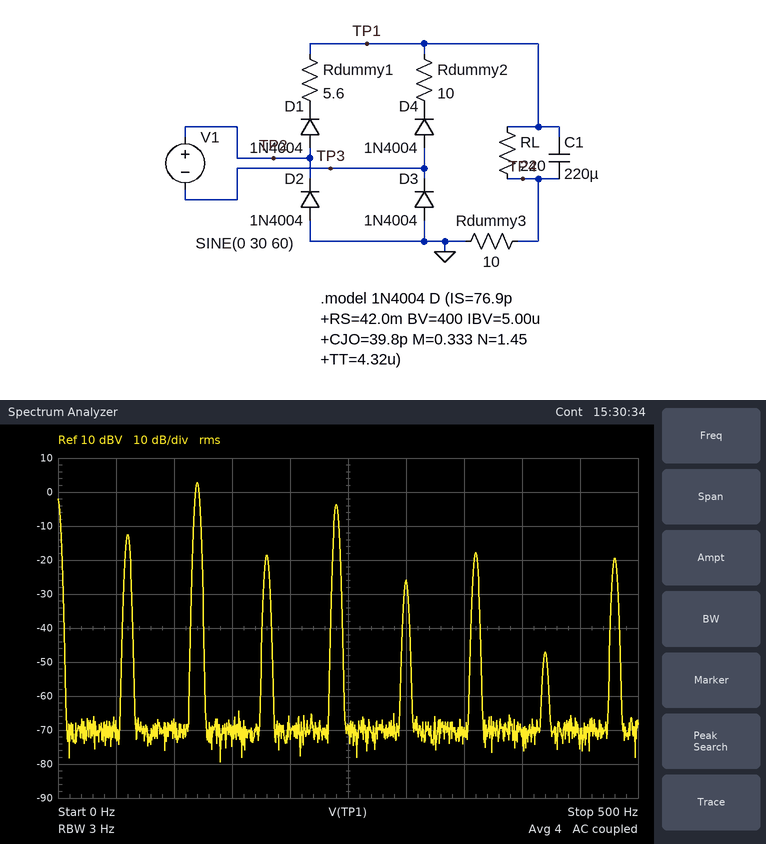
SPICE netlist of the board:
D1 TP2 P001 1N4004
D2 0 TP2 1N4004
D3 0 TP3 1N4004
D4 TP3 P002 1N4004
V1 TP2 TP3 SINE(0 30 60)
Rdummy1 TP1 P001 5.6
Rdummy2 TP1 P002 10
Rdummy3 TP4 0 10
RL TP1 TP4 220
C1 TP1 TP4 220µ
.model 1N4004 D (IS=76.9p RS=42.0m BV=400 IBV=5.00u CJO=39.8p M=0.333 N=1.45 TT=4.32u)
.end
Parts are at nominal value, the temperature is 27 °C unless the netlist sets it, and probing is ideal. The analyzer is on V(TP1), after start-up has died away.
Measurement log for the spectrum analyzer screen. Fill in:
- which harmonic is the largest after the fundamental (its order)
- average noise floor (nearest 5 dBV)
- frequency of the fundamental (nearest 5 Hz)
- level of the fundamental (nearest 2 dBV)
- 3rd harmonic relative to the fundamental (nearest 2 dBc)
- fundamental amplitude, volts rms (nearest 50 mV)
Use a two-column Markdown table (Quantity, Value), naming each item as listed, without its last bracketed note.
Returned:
| Quantity | Value |
|---|---|
| which harmonic is the largest after the fundamental | 2 |
| average noise floor | -70 dBV |
| frequency of the fundamental | 60 Hz |
| level of the fundamental | -12 dBV |
| 3rd harmonic relative to the fundamental | -6 dBc |
| fundamental amplitude, volts rms | 250 mV |
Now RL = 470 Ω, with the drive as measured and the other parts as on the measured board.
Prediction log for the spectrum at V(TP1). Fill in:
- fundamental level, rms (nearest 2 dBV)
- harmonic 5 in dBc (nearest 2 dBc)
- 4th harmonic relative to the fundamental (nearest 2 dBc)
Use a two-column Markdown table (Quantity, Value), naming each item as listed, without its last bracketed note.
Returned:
| Quantity | Value |
|---|---|
| fundamental level, rms | -18 dBV |
| harmonic 5 in dBc | -10 dBc |
| 4th harmonic relative to the fundamental | 12 dBc |
